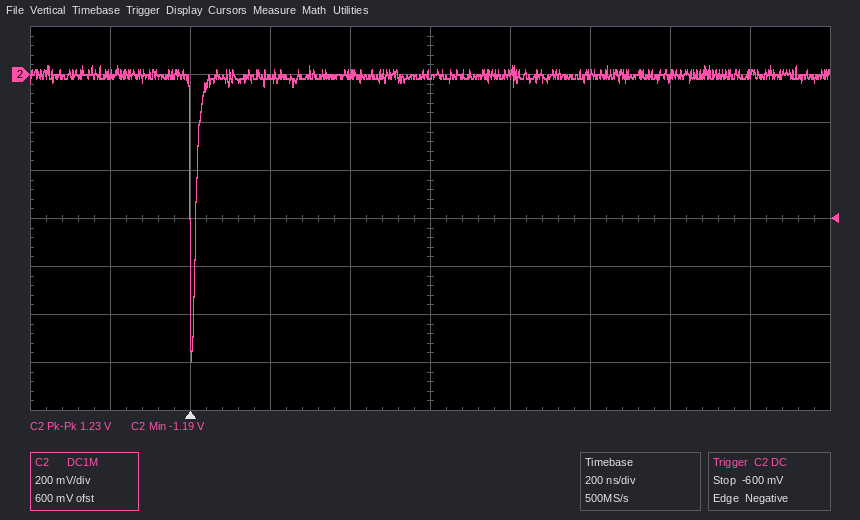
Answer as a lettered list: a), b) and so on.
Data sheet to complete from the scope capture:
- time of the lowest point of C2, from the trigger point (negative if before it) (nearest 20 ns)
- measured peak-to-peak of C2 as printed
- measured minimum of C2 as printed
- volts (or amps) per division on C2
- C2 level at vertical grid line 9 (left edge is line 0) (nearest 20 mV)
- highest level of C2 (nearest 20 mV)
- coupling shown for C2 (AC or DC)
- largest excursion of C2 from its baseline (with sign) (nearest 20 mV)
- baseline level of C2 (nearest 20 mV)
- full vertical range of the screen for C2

a) 0 ns
b) 1.23 V
c) -1.19 V
d) 200 mV
e) 0 mV
f) 40 mV
g) DC
h) -1.18 V
i) 0 mV
j) 1.6 V
